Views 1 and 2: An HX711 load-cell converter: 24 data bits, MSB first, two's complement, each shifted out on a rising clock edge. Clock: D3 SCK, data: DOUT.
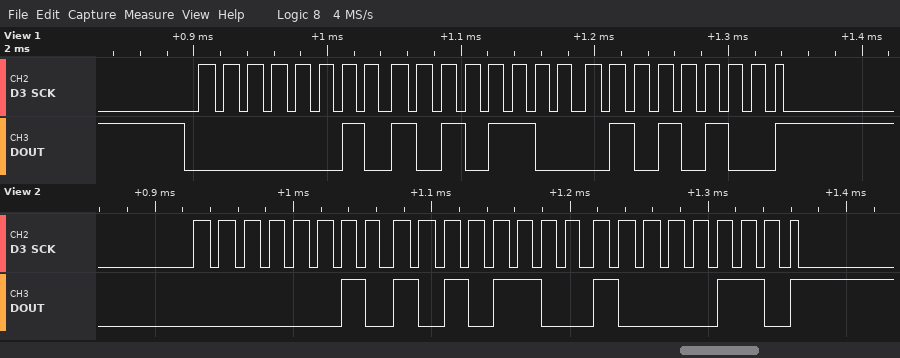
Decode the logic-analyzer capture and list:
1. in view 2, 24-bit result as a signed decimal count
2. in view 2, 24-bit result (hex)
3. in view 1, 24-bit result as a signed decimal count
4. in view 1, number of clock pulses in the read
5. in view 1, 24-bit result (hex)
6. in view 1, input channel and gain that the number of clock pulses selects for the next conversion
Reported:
175238
0x02AC86
175188
25
0x02AC54
channel A, gain 128
